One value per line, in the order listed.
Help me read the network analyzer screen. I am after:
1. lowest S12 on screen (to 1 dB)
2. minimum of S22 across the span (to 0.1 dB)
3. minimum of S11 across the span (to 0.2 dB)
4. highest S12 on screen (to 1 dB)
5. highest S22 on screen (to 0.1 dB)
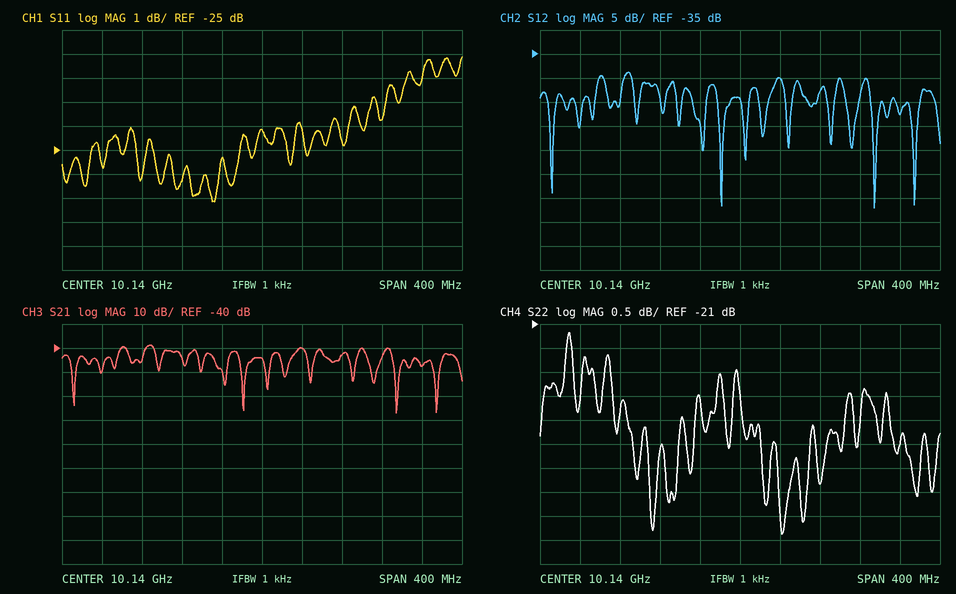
-67 dB
-25.4 dB
-27.2 dB
-39 dB
-21.2 dB
